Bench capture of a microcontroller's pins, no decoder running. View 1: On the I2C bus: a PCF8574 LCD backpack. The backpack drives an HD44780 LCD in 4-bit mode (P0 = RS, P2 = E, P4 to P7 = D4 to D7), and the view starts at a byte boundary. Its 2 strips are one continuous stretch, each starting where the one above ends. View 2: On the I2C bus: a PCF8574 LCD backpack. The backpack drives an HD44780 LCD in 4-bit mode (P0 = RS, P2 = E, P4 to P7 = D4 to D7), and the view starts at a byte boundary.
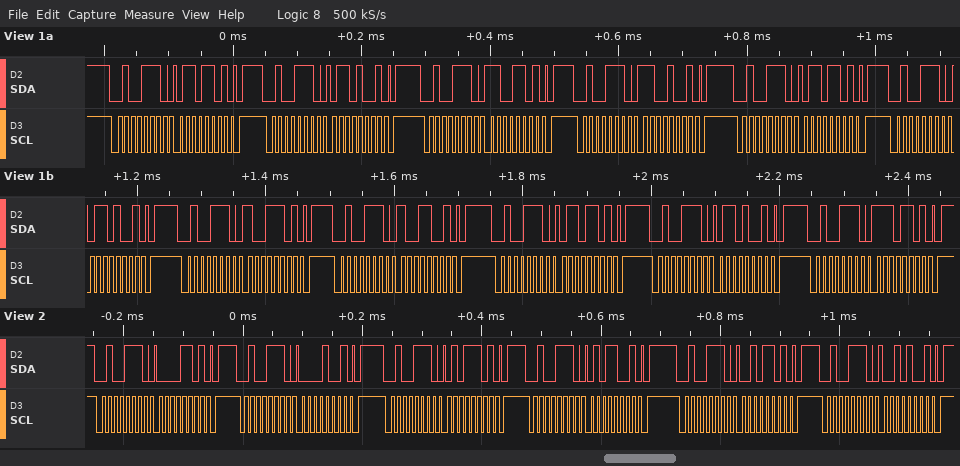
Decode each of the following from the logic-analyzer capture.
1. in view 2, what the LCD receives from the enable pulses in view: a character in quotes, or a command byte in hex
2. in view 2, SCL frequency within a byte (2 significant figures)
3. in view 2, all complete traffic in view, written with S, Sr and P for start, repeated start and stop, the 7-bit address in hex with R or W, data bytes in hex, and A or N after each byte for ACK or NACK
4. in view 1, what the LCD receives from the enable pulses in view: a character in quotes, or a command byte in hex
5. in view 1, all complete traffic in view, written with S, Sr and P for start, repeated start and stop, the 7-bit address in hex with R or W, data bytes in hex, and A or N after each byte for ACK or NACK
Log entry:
data 0x05
100 kHz
S 27W A 0D A P S 27W A 09 A P S 27W A 5D A P S 27W A 59 A P S 27W A 2D A P S 27W A 29 A P
'l' 'i'
S 27W A 6D A P S 27W A 69 A P S 27W A CD A P S 27W A C9 A P S 27W A 6D A P S 27W A 69 A P S 27W A 9D A P S 27W A 99 A P S 27W A 6D A P S 27W A 69 A P S 27W A ED A P
